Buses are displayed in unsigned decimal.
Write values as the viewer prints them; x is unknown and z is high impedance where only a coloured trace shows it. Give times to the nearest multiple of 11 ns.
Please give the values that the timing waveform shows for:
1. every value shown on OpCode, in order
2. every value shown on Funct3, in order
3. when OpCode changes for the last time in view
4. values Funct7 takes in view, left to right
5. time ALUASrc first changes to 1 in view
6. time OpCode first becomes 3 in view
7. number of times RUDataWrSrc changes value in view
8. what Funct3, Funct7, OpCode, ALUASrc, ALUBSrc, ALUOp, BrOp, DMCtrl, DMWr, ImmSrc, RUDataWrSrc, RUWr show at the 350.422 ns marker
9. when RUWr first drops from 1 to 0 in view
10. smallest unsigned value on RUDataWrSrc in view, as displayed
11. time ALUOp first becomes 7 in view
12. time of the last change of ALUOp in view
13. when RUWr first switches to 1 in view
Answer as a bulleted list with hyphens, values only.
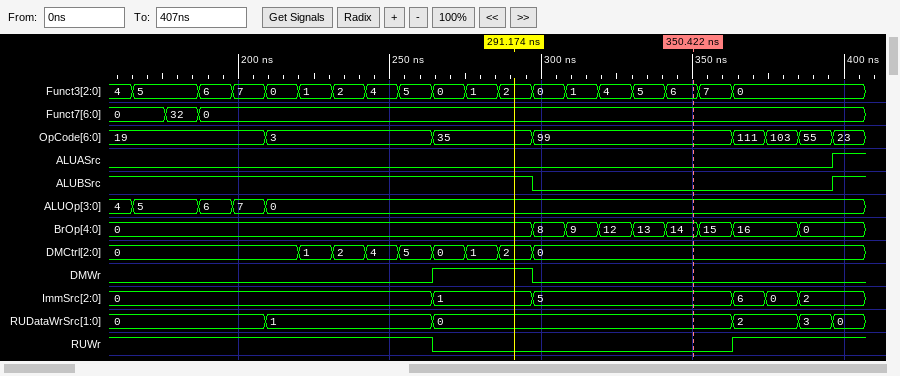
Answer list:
- 19, 3, 35, 99, 111, 103, 55, 23
- 4, 5, 6, 7, 0, 1, 2, 4, 5, 0, 1, 2, 0, 1, 4, 5, 6, 7, 0
- 396 ns
- 0, 32, 0
- 396 ns
- 209 ns
- 5
- Funct3=6, Funct7=0, OpCode=99, ALUASrc=0, ALUBSrc=0, ALUOp=0, BrOp=14, DMCtrl=0, DMWr=0, ImmSrc=5, RUDataWrSrc=0, RUWr=0
- 264 ns
- 0
- 198 ns
- 209 ns
- 363 ns
